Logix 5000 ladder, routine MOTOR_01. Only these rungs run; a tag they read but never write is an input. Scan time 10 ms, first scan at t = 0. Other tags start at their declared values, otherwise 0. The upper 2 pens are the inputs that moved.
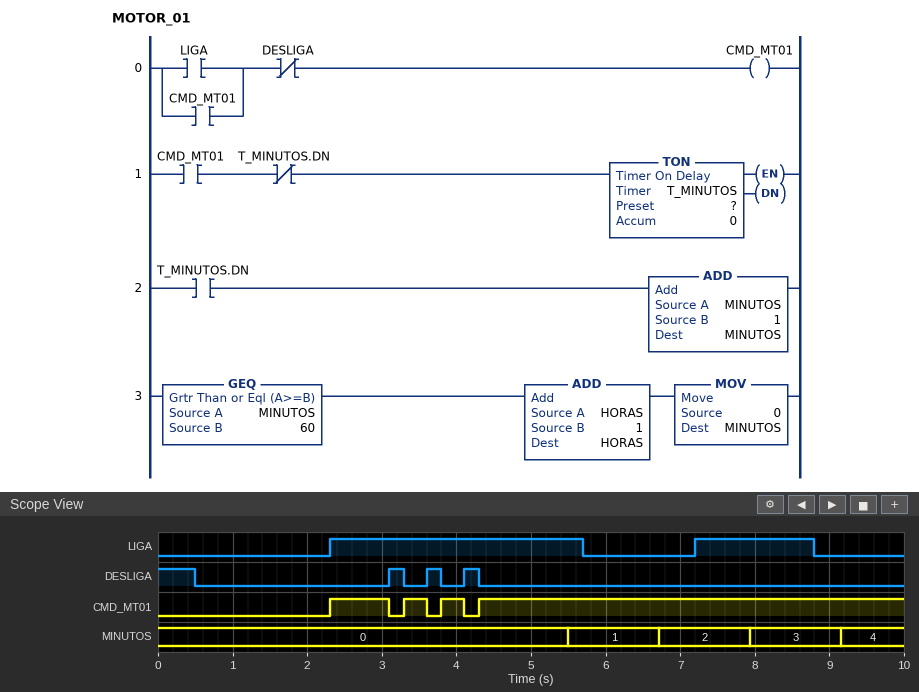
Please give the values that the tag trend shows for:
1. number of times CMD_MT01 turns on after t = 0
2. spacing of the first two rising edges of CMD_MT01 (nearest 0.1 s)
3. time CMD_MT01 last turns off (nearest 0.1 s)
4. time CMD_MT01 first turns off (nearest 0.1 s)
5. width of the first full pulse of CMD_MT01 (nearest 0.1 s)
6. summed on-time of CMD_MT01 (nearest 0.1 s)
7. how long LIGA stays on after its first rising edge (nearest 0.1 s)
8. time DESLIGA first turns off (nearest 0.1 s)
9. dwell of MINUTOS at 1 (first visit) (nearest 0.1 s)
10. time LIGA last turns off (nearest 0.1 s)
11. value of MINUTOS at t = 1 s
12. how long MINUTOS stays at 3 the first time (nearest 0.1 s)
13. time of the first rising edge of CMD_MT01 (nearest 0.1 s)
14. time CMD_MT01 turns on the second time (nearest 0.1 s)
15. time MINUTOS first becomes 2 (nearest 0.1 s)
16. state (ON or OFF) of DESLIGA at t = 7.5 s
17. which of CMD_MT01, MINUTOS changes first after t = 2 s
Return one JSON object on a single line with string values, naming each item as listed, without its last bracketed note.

{"number of times CMD_MT01 turns on after t = 0": "4", "spacing of the first two rising edges of CMD_MT01": "1.0 s", "time CMD_MT01 last turns off": "4.1 s", "time CMD_MT01 first turns off": "3.1 s", "width of the first full pulse of CMD_MT01": "0.8 s", "summed on-time of CMD_MT01": "7.1 s", "how long LIGA stays on after its first rising edge": "3.4 s", "time DESLIGA first turns off": "0.5 s", "dwell of MINUTOS at 1 (first visit)": "1.2 s", "time LIGA last turns off": "8.8 s", "value of MINUTOS at t = 1 s": "0", "how long MINUTOS stays at 3 the first time": "1.2 s", "time of the first rising edge of CMD_MT01": "2.3 s", "time CMD_MT01 turns on the second time": "3.3 s", "time MINUTOS first becomes 2": "6.7 s", "state (ON or OFF) of DESLIGA at t = 7.5 s": "OFF", "which of CMD_MT01, MINUTOS changes first after t = 2 s": "CMD_MT01"}
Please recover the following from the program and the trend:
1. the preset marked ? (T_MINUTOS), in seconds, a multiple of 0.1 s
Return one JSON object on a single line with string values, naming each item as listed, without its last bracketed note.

{"the preset marked ? (T_MINUTOS), in seconds, a multiple of 0.1 s": "1.2 s"}
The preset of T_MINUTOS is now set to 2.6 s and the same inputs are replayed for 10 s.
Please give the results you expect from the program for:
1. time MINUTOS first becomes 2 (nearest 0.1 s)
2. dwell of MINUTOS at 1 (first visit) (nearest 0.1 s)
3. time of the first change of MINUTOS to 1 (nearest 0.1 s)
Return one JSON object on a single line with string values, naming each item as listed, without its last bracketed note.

{"time MINUTOS first becomes 2": "9.5 s", "dwell of MINUTOS at 1 (first visit)": "2.6 s", "time of the first change of MINUTOS to 1": "6.9 s"}
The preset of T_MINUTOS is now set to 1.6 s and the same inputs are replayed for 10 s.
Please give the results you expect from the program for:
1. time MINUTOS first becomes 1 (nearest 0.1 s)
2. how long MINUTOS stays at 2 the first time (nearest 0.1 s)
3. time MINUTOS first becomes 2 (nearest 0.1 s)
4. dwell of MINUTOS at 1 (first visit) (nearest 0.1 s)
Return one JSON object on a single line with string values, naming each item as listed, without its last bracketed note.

{"time MINUTOS first becomes 1": "5.9 s", "how long MINUTOS stays at 2 the first time": "1.6 s", "time MINUTOS first becomes 2": "7.5 s", "dwell of MINUTOS at 1 (first visit)": "1.6 s"}
